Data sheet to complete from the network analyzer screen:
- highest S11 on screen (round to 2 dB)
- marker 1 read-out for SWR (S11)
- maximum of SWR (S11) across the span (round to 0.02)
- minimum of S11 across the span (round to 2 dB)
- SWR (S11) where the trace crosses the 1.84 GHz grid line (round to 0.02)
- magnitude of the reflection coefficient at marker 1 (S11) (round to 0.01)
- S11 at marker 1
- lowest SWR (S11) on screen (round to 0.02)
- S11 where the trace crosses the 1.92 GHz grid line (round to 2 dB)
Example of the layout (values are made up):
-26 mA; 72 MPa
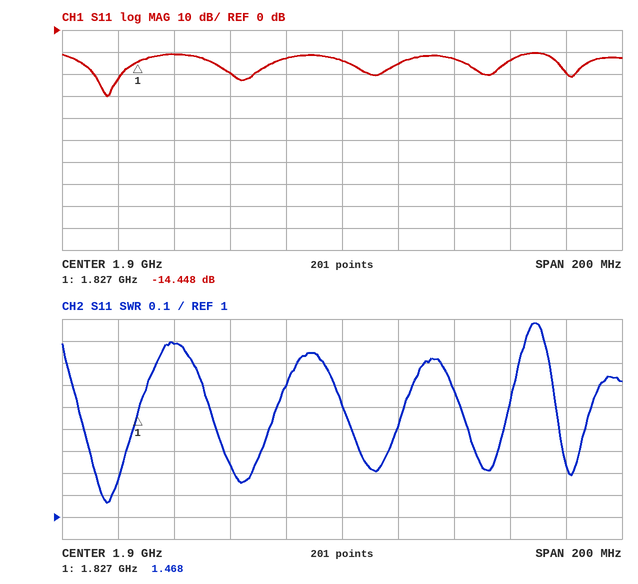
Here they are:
-10 dB; 1.468; 1.88; -30 dB; 1.78; 0.19; -14.448 dB; 1.06; -16 dB
